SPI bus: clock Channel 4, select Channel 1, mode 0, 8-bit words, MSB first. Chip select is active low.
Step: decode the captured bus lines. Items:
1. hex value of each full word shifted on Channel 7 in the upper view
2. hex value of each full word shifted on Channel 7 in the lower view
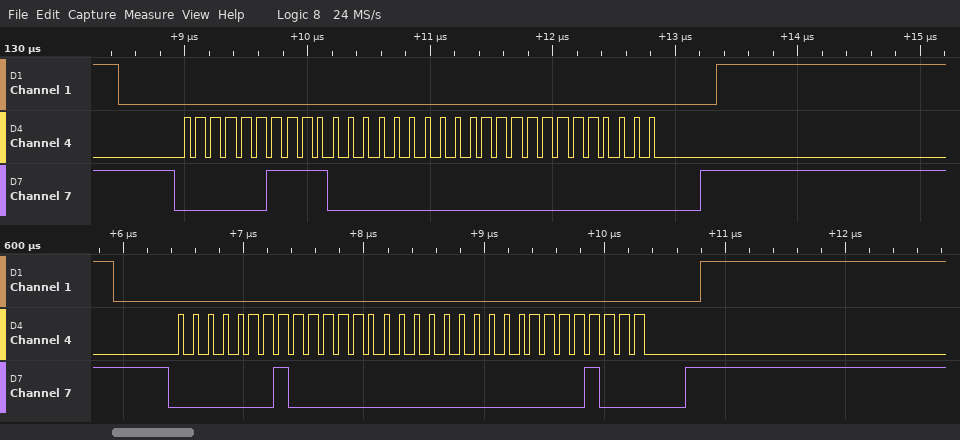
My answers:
03, C0, 00, 00
01, 00, 00, 08
